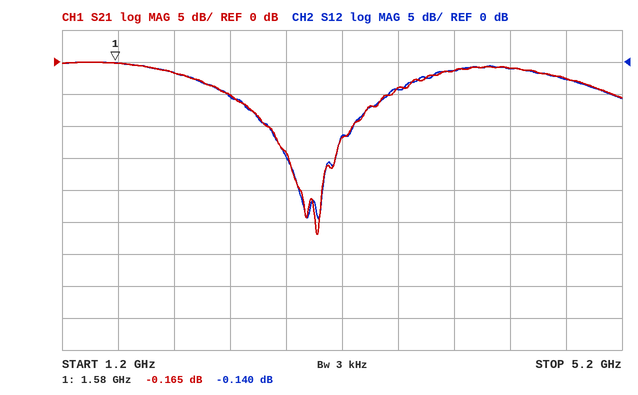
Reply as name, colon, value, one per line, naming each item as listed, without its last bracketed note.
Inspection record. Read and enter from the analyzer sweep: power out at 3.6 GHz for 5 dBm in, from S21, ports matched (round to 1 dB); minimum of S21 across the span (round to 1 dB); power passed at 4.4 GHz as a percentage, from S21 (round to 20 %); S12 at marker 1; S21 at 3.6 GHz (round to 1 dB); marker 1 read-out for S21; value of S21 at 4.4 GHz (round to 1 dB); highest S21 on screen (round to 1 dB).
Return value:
power out at 3.6 GHz for 5 dBm in, from S21, ports matched: 1 dBm
minimum of S21 across the span: -27 dB
power passed at 4.4 GHz as a percentage, from S21: 80 %
S12 at marker 1: -0.140 dB
S21 at 3.6 GHz: -4 dB
marker 1 read-out for S21: -0.165 dB
value of S21 at 4.4 GHz: -1 dB
highest S21 on screen: 0 dB
